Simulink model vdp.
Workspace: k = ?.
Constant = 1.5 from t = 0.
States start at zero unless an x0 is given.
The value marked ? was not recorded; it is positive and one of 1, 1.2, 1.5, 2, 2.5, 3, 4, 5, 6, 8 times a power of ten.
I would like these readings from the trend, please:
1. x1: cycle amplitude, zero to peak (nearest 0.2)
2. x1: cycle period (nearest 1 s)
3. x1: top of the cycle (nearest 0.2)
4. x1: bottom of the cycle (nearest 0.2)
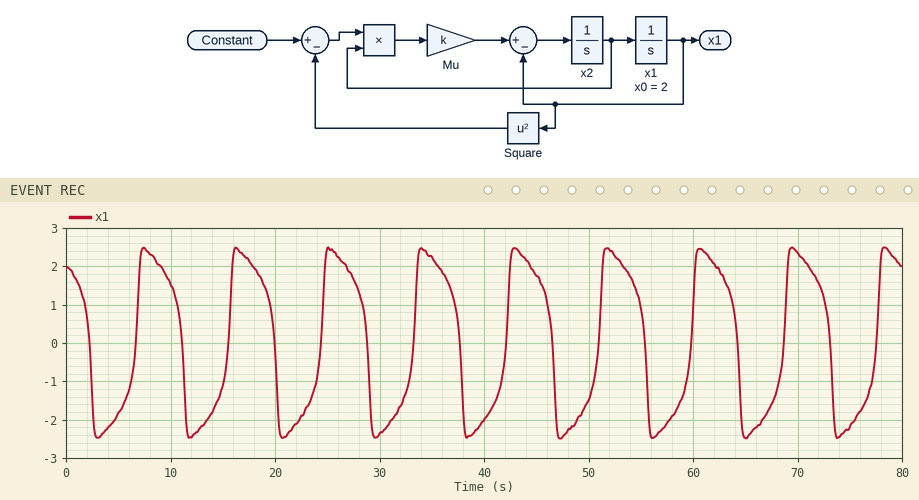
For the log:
2.4
9 s
2.4
-2.4
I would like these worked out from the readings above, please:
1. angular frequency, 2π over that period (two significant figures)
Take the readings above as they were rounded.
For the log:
0.70 rad/s
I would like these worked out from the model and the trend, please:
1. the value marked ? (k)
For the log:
2
